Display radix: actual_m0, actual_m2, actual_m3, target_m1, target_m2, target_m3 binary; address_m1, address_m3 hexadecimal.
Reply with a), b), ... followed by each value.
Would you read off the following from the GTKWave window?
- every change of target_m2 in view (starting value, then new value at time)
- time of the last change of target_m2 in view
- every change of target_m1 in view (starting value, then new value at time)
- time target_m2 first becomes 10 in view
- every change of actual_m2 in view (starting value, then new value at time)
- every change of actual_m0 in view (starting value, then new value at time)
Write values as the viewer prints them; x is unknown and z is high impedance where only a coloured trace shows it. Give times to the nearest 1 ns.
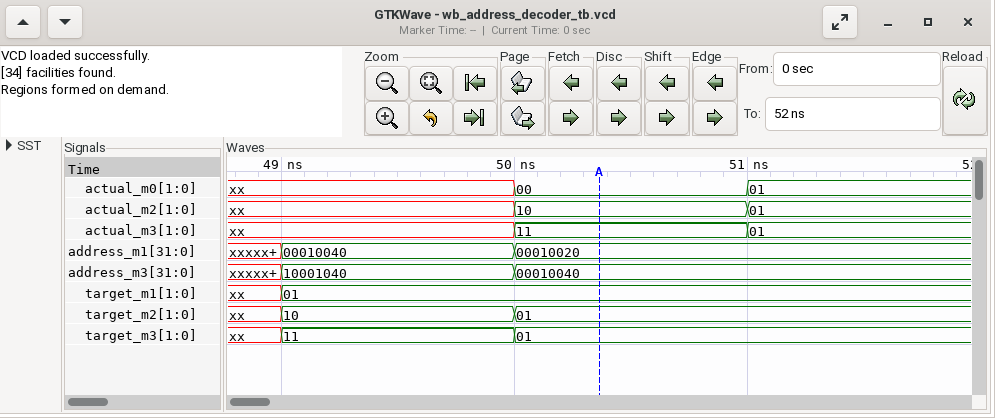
a) xx, 10 at 49 ns, 01 at 50 ns
b) 50 ns
c) xx, 01 at 49 ns
d) 49 ns
e) xx, 10 at 50 ns, 01 at 51 ns
f) xx, 00 at 50 ns, 01 at 51 ns
